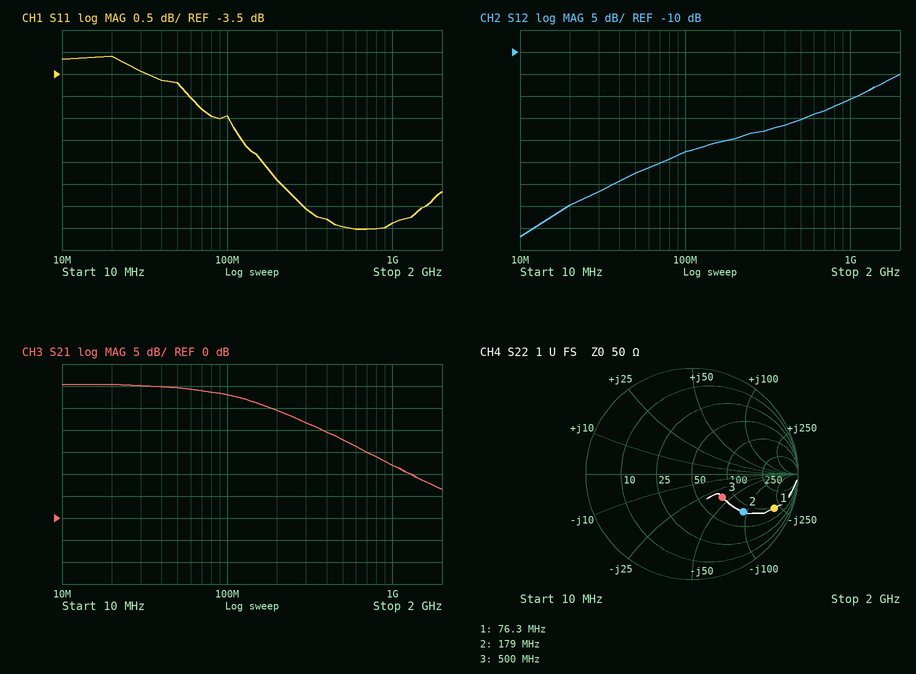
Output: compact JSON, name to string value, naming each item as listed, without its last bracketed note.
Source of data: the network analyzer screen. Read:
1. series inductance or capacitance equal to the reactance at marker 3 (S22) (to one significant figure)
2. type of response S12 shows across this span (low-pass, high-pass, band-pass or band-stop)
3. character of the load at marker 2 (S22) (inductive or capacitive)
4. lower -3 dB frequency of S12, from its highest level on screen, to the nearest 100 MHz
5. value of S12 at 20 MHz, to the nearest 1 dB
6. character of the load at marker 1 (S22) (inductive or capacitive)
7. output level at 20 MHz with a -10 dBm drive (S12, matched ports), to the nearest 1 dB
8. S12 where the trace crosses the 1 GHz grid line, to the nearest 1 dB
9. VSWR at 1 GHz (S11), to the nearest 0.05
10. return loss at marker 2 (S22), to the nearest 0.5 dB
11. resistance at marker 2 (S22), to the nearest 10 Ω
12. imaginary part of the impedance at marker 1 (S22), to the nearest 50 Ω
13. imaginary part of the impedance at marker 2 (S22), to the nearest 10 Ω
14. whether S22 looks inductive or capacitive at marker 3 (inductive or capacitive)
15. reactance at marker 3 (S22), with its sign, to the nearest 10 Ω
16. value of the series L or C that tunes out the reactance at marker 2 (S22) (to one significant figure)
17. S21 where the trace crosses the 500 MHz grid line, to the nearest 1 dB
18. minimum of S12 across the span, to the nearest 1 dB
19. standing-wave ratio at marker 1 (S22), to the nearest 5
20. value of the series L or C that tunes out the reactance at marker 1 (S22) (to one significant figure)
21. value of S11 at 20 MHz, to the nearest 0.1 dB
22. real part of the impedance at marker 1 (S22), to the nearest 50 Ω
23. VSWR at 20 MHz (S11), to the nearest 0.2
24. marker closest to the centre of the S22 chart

{"series inductance or capacitance equal to the reactance at marker 3 (S22)": "8 pF", "type of response S12 shows across this span": "high-pass", "character of the load at marker 2 (S22)": "capacitive", "lower -3 dB frequency of S12, from its highest level on screen, to the nearest 100 MHz": "1.4 GHz", "value of S12 at 20 MHz, to the nearest 1 dB": "-45 dB", "character of the load at marker 1 (S22)": "capacitive", "output level at 20 MHz with a -10 dBm drive (S12, matched ports), to the nearest 1 dB": "-55 dBm", "S12 where the trace crosses the 1 GHz grid line, to the nearest 1 dB": "-21 dB", "VSWR at 1 GHz (S11), to the nearest 0.05": "2.65", "return loss at marker 2 (S22), to the nearest 0.5 dB": "4.5 dB", "resistance at marker 2 (S22), to the nearest 10 Ω": "80 Ω", "imaginary part of the impedance at marker 1 (S22), to the nearest 50 Ω": "-200 Ω", "imaginary part of the impedance at marker 2 (S22), to the nearest 10 Ω": "-90 Ω", "whether S22 looks inductive or capacitive at marker 3": "capacitive", "reactance at marker 3 (S22), with its sign, to the nearest 10 Ω": "-40 Ω", "value of the series L or C that tunes out the reactance at marker 2 (S22)": "80 nH", "S21 where the trace crosses the 500 MHz grid line, to the nearest 1 dB": "18 dB", "minimum of S12 across the span, to the nearest 1 dB": "-52 dB", "standing-wave ratio at marker 1 (S22), to the nearest 5": "10", "value of the series L or C that tunes out the reactance at marker 1 (S22)": "400 nH", "value of S11 at 20 MHz, to the nearest 0.1 dB": "-3.1 dB", "real part of the impedance at marker 1 (S22), to the nearest 50 Ω": "100 Ω", "VSWR at 20 MHz (S11), to the nearest 0.2": "5.6", "marker closest to the centre of the S22 chart": "marker 3"}
